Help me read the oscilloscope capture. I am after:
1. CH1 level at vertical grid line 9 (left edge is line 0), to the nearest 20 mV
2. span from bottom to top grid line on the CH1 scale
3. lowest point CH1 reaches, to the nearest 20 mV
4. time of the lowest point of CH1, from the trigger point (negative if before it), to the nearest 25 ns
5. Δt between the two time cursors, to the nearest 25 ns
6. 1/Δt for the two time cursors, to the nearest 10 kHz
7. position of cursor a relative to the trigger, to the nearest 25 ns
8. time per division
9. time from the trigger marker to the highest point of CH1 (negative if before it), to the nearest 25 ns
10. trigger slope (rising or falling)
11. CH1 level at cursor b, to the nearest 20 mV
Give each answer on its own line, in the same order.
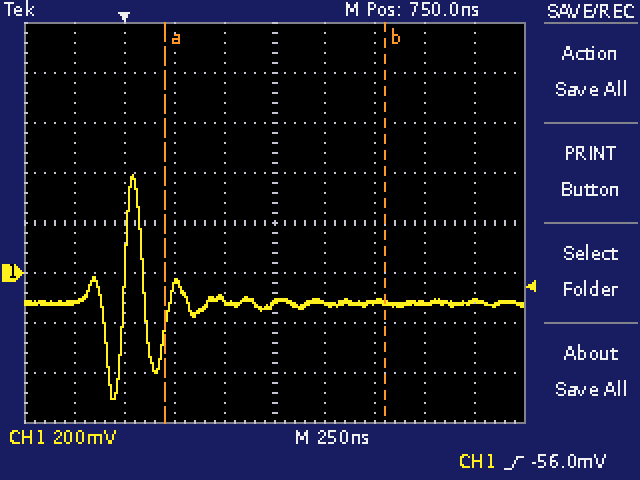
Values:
-120 mV
1.6 V
-500 mV
-50 ns
1.100 µs
910 kHz
+200 ns
250 ns
+50 ns
rising
-120 mV
